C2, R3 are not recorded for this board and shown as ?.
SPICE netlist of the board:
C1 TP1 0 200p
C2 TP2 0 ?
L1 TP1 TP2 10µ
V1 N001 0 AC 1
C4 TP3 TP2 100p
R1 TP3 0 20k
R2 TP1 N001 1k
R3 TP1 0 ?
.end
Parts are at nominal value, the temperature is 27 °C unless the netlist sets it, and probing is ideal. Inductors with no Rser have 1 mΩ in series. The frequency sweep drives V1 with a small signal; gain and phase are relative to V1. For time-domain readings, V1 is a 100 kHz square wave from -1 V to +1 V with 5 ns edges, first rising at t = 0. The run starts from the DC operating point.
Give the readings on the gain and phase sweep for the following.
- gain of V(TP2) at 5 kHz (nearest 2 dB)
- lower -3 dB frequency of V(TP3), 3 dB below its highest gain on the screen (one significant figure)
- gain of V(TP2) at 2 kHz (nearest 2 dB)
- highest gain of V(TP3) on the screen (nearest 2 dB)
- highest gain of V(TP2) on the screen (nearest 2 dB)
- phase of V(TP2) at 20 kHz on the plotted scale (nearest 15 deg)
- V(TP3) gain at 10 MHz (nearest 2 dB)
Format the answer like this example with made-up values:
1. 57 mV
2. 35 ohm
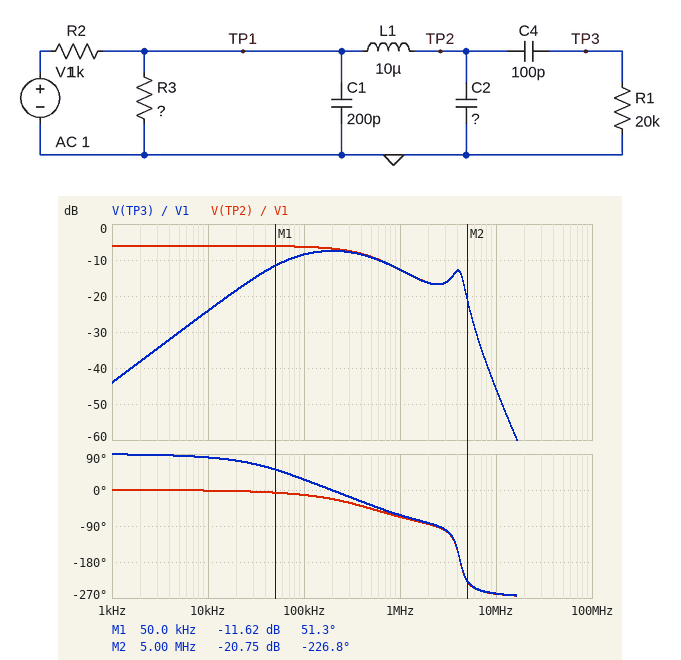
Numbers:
1. -6 dB
2. 60 kHz
3. -6 dB
4. -8 dB
5. -6 dB
6. 0 deg
7. -46 dB
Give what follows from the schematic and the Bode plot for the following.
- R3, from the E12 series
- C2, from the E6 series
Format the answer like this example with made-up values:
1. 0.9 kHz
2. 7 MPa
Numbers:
1. 1 kΩ
2. 470 pF
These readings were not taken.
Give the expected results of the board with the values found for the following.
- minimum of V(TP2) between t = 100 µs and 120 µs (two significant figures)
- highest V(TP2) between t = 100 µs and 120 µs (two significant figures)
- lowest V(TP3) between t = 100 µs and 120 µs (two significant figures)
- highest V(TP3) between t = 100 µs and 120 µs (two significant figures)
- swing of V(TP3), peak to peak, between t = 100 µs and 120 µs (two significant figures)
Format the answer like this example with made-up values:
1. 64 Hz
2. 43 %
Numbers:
1. -500 mV
2. 500 mV
3. -640 mV
4. 640 mV
5. 1.3 V
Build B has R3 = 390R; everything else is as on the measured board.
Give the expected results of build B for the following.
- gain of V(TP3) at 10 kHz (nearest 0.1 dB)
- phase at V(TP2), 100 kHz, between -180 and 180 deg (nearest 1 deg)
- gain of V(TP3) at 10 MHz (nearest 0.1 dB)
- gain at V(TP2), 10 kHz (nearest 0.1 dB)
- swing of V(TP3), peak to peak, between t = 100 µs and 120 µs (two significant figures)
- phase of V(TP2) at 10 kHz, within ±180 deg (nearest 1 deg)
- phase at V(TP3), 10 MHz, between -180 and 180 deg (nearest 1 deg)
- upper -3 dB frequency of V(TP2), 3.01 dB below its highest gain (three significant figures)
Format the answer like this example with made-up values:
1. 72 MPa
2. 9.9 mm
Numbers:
1. -29.1 dB
2. -7 deg
3. -46.1 dB
4. -11.0 dB
5. 830 mV
6. -1 deg
7. 109 deg
8. 1.04 MHz
